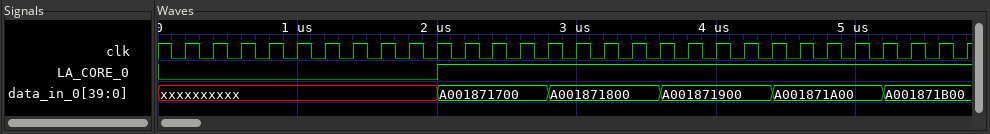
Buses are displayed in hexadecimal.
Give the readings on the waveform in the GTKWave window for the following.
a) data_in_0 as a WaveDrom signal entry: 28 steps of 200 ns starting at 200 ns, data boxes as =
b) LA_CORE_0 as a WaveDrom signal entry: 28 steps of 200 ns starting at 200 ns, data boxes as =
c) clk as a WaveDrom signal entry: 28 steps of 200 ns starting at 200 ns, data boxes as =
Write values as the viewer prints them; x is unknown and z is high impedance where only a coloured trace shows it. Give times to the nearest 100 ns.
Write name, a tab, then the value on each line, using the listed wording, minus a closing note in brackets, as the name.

data_in_0 as a WaveDrom signal entry: 28 steps of 200 ns starting at 200 ns, data boxes as =	{name: 'data_in_0', wave: 'x........=...=...=...=...=..', data: 'A001871700 A001871800 A001871900 A001871A00 A001871B00'}
LA_CORE_0 as a WaveDrom signal entry: 28 steps of 200 ns starting at 200 ns, data boxes as =	{name: 'LA_CORE_0', wave: '0........1..................'}
clk as a WaveDrom signal entry: 28 steps of 200 ns starting at 200 ns, data boxes as =	{name: 'clk', wave: 'p...........................'}
